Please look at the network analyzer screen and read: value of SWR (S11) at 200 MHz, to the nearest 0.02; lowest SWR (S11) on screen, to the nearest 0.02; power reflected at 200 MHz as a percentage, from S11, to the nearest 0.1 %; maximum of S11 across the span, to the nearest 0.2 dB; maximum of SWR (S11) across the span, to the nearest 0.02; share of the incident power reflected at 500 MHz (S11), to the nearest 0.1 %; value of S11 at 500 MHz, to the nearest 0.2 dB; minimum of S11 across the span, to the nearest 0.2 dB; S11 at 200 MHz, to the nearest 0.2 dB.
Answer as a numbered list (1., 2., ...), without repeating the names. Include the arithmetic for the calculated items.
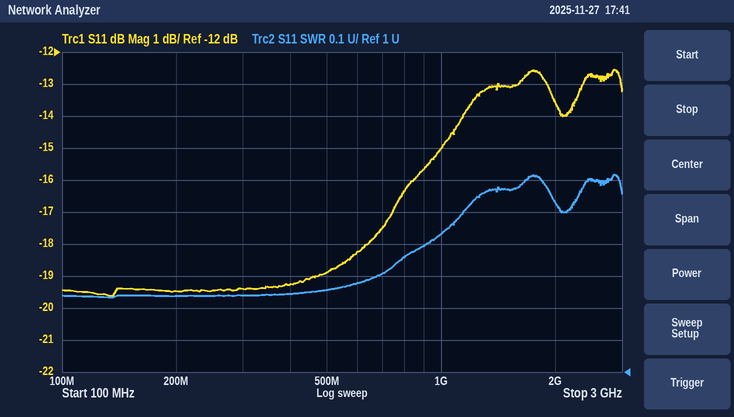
1. 1.24
2. 1.24
3. 10^(-19.4/10) ≈ 1.1 %
4. -12.6 dB
5. 1.62
6. 10^(-18.8/10) ≈ 1.3 %
7. -18.8 dB
8. -19.6 dB
9. -19.4 dB
